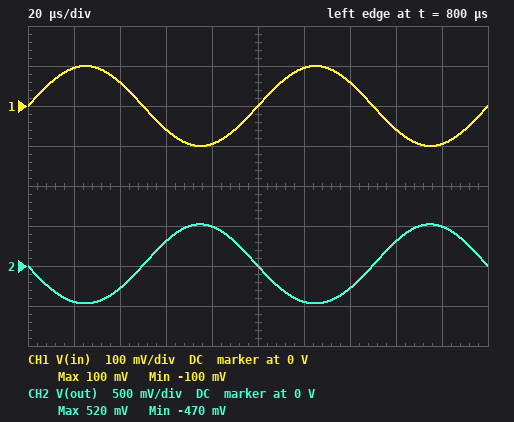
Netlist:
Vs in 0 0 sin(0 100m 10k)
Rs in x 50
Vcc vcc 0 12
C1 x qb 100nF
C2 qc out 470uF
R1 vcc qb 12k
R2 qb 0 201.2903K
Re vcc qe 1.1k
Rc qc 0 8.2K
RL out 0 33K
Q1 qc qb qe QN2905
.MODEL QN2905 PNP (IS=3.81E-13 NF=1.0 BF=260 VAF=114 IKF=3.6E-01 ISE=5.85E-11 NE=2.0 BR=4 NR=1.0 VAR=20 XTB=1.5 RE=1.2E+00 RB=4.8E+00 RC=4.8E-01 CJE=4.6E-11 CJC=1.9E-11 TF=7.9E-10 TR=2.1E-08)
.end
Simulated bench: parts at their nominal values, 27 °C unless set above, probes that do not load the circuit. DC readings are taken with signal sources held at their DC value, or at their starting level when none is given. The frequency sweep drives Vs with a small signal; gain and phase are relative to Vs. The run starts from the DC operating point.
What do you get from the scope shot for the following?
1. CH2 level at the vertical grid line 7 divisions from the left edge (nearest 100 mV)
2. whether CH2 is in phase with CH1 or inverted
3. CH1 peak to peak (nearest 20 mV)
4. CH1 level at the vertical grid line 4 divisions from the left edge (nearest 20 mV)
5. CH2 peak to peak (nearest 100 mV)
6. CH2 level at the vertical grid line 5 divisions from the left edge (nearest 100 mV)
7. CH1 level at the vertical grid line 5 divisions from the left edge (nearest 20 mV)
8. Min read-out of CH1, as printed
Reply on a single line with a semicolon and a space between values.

-300 mV; inverted; 200 mV; -100 mV; 1.0 V; 0 V; 0 V; -100 mV
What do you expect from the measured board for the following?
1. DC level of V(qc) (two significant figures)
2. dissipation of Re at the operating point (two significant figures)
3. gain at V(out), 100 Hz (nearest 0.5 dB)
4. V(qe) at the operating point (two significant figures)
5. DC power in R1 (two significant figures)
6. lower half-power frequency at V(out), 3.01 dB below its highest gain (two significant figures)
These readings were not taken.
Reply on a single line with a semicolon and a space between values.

1.1 V; 20 µW; 9.0 dB; 12 V; 36 µW; 150 Hz
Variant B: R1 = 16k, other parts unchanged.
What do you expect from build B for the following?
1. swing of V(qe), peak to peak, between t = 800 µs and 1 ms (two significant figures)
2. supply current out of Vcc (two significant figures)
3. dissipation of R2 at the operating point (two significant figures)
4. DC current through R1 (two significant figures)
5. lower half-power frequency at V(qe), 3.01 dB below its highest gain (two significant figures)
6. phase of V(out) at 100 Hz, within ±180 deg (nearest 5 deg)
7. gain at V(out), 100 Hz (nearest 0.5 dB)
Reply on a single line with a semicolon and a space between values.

180 mV; 340 µA; 620 µW; 53 µA; 120 Hz; -130 deg; 11.0 dB
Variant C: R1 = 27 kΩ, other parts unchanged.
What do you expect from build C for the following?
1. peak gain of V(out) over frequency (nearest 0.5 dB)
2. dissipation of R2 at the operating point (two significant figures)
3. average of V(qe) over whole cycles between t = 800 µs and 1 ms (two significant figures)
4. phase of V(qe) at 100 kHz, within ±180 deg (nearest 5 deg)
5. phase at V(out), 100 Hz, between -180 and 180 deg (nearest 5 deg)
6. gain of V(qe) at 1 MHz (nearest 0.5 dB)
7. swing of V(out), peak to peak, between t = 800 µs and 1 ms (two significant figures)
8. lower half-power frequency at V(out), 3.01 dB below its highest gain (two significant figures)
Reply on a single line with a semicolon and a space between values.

15.0 dB; 570 µW; 11 V; 0 deg; -145 deg; -0.5 dB; 1.1 V; 75 Hz
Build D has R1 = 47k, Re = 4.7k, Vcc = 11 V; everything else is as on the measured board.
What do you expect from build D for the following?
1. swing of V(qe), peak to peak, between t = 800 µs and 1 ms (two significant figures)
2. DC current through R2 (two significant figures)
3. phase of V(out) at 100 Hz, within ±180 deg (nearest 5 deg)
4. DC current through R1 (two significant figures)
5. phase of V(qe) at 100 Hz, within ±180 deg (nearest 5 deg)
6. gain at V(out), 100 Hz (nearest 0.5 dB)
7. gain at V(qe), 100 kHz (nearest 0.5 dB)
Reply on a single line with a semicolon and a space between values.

200 mV; 45 µA; -155 deg; 42 µA; 25 deg; 2.0 dB; 0 dB
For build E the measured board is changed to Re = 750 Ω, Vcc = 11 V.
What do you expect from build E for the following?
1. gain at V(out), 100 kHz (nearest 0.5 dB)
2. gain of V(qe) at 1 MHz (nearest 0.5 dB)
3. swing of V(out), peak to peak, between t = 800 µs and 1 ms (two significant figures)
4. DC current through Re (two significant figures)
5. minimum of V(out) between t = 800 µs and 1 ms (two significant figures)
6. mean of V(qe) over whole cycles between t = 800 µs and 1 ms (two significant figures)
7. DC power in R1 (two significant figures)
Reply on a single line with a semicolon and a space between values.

16.5 dB; -2.0 dB; 1.3 V; 130 µA; -580 mV; 11 V; 30 µW
